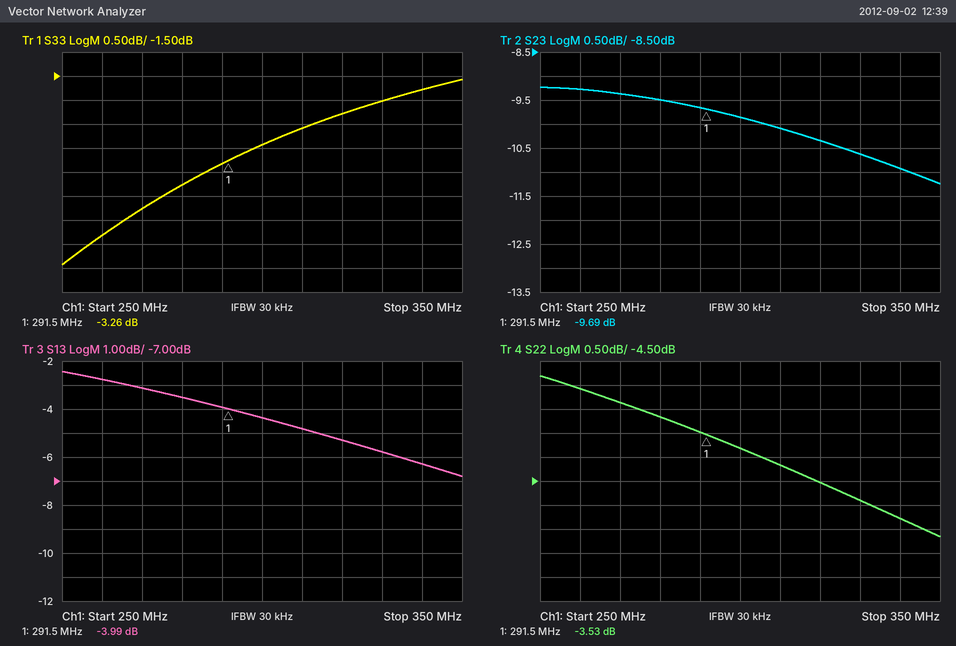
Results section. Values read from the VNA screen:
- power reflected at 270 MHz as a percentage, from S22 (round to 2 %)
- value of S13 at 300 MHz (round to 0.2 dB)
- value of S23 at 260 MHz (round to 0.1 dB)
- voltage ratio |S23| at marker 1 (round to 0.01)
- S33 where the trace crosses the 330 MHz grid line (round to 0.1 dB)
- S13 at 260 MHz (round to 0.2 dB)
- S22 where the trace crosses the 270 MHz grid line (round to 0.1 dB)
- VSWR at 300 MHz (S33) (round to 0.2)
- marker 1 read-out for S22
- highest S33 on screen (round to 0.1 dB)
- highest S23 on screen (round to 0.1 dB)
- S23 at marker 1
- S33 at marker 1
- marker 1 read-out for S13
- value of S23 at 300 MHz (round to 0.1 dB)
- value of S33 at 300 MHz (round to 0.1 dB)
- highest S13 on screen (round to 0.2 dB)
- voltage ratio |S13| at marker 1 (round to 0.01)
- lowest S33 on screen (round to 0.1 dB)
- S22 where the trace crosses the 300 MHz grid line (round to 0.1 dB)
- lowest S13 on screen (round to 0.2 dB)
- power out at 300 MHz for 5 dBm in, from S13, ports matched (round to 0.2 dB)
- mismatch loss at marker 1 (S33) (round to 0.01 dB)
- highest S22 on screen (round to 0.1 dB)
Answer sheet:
52 %
-4.4 dB
-9.3 dB
0.33
-2.0 dB
-2.8 dB
-2.9 dB
6.0
-3.53 dB
-1.6 dB
-9.2 dB
-9.69 dB
-3.26 dB
-3.99 dB
-9.9 dB
-2.9 dB
-2.4 dB
0.63
-5.4 dB
-3.8 dB
-6.8 dB
0.6 dBm
2.77 dB
-2.3 dB
